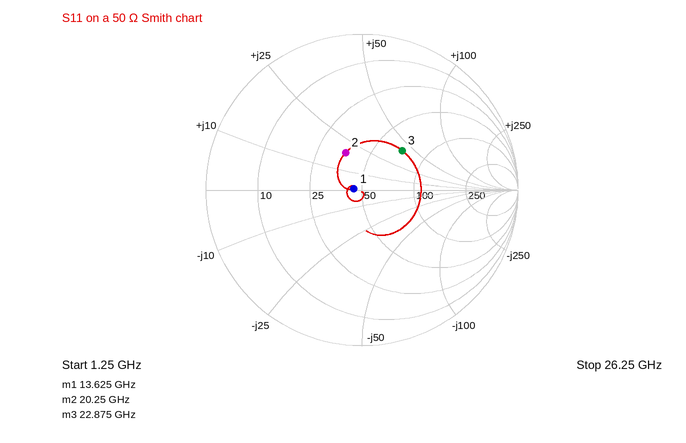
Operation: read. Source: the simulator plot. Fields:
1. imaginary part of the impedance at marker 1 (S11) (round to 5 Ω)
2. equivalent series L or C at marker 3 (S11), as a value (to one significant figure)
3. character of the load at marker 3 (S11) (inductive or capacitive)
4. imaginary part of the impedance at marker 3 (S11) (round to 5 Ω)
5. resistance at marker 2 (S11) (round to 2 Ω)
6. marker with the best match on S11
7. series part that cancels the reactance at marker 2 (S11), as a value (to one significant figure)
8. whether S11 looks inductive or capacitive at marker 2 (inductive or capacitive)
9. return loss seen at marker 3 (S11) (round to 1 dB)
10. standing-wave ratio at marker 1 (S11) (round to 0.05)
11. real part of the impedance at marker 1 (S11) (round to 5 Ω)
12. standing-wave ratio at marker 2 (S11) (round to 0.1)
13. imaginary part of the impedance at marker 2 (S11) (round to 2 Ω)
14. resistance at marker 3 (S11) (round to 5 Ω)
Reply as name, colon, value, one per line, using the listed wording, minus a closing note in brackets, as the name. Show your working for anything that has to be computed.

imaginary part of the impedance at marker 1 (S11): 0 Ω
equivalent series L or C at marker 3 (S11), as a value: L = 40 Ω/(2π × 22.875 GHz) ≈ 278 pH, so 300 pH to one significant figure
character of the load at marker 3 (S11): inductive
imaginary part of the impedance at marker 3 (S11): +40 Ω
resistance at marker 2 (S11): 36 Ω
marker with the best match on S11: marker 1
series part that cancels the reactance at marker 2 (S11), as a value: C = 1/(2π × 20.25 GHz × 18 Ω) ≈ 437 fF, so 400 fF to one significant figure
whether S11 looks inductive or capacitive at marker 2: inductive
return loss seen at marker 3 (S11): 9 dB
standing-wave ratio at marker 1 (S11): 1.10
real part of the impedance at marker 1 (S11): 45 Ω
standing-wave ratio at marker 2 (S11): 1.7
imaginary part of the impedance at marker 2 (S11): +18 Ω
resistance at marker 3 (S11): 70 Ω
